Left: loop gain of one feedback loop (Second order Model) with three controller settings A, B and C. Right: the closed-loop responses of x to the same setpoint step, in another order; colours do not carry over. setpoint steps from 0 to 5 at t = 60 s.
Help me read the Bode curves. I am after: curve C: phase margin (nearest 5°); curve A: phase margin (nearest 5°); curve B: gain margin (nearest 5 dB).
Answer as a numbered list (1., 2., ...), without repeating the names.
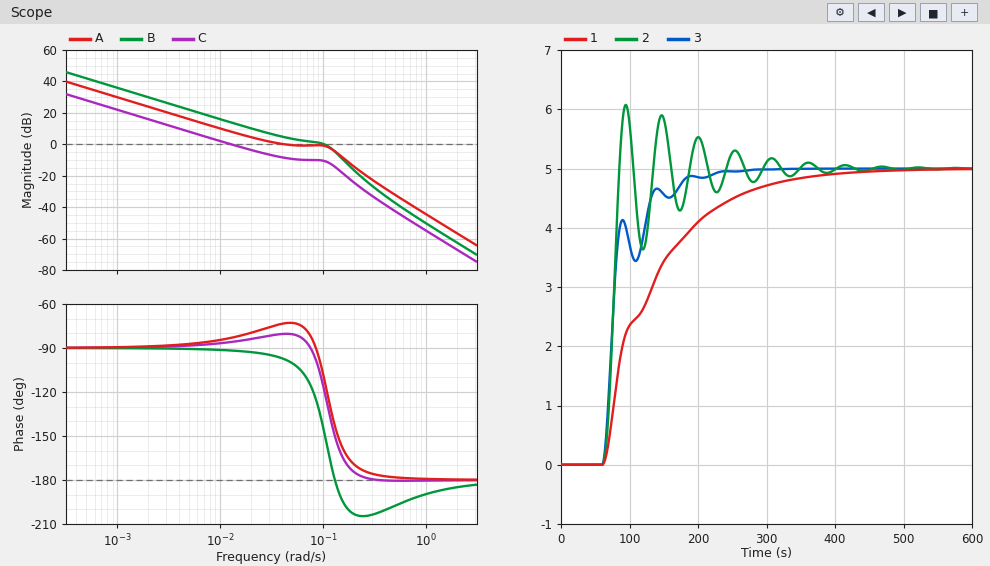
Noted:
1. 95°
2. 105°
3. 5 dB
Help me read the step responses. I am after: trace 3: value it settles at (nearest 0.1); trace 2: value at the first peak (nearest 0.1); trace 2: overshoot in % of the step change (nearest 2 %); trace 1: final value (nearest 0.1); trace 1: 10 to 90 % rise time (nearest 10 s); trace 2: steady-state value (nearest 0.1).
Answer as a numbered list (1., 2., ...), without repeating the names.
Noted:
1. 5.0
2. 6.1
3. 22 %
4. 5.0
5. 180 s
6. 5.0
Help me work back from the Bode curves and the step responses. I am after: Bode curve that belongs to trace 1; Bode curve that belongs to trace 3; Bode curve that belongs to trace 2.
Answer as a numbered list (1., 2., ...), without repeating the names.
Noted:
1. C
2. A
3. B
